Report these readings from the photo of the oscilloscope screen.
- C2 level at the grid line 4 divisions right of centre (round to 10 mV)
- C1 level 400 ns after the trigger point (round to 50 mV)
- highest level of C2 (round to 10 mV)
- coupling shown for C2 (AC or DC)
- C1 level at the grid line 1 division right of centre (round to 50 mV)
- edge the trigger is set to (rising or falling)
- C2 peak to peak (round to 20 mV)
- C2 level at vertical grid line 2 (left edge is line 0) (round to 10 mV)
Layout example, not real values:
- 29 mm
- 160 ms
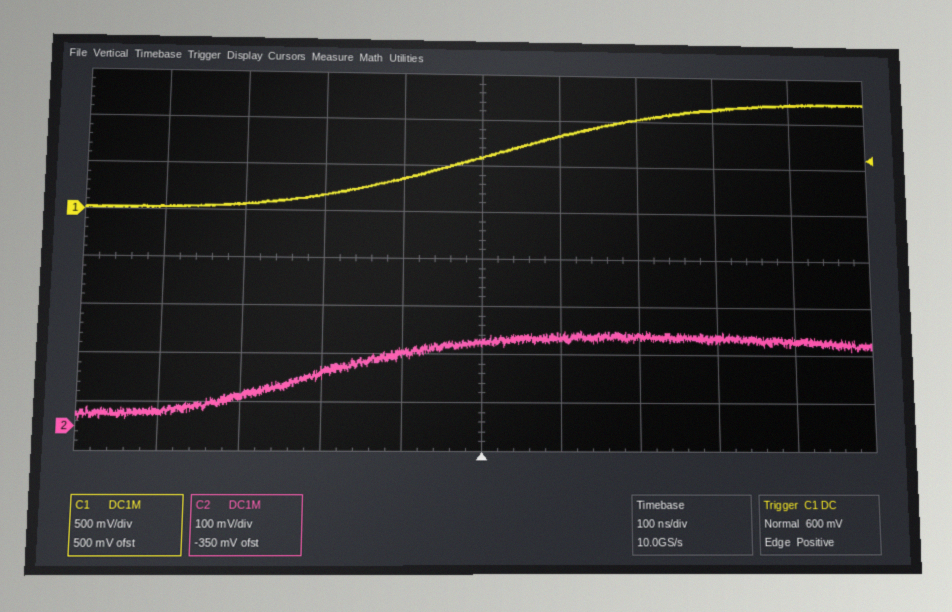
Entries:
- 180 mV
- 1.20 V
- 200 mV
- DC
- 850 mV
- rising
- 180 mV
- 60 mV
